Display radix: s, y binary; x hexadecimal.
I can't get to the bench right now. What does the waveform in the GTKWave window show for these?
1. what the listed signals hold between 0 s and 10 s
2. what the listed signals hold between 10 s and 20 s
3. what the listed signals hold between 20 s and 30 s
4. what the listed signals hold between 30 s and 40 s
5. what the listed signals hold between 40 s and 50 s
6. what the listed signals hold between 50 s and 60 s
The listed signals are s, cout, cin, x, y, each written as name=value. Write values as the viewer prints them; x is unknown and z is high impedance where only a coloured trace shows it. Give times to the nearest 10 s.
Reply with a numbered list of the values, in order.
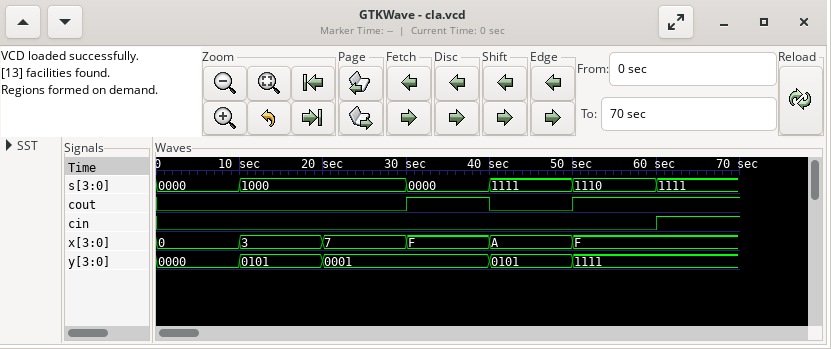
1. s=0000, cout=0, cin=0, x=0, y=0000
2. s=1000, cout=0, cin=0, x=3, y=0101
3. s=1000, cout=0, cin=0, x=7, y=0001
4. s=0000, cout=1, cin=0, x=F, y=0001
5. s=1111, cout=0, cin=0, x=A, y=0101
6. s=1110, cout=1, cin=0, x=F, y=1111
